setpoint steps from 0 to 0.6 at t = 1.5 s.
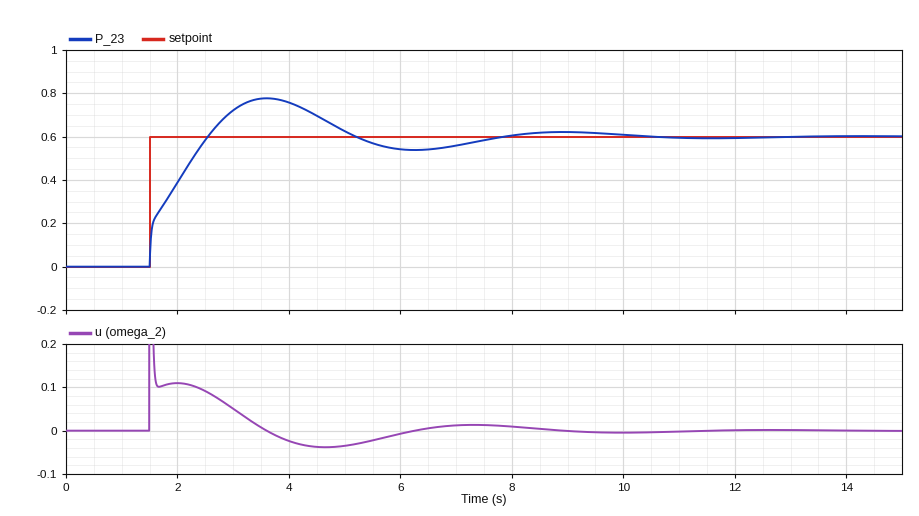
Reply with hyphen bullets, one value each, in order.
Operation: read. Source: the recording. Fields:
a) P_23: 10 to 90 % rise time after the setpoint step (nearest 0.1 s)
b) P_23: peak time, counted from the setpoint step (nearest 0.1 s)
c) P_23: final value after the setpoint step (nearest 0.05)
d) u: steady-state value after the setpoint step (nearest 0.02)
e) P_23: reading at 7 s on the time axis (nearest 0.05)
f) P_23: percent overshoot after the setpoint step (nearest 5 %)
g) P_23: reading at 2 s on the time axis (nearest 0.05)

- 0.9 s
- 2.1 s
- 0.60
- 0.00
- 0.55
- 30 %
- 0.40
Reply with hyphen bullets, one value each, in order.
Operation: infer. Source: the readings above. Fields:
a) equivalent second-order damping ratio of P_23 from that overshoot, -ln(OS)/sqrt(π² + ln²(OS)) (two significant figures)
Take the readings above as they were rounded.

- 0.36
